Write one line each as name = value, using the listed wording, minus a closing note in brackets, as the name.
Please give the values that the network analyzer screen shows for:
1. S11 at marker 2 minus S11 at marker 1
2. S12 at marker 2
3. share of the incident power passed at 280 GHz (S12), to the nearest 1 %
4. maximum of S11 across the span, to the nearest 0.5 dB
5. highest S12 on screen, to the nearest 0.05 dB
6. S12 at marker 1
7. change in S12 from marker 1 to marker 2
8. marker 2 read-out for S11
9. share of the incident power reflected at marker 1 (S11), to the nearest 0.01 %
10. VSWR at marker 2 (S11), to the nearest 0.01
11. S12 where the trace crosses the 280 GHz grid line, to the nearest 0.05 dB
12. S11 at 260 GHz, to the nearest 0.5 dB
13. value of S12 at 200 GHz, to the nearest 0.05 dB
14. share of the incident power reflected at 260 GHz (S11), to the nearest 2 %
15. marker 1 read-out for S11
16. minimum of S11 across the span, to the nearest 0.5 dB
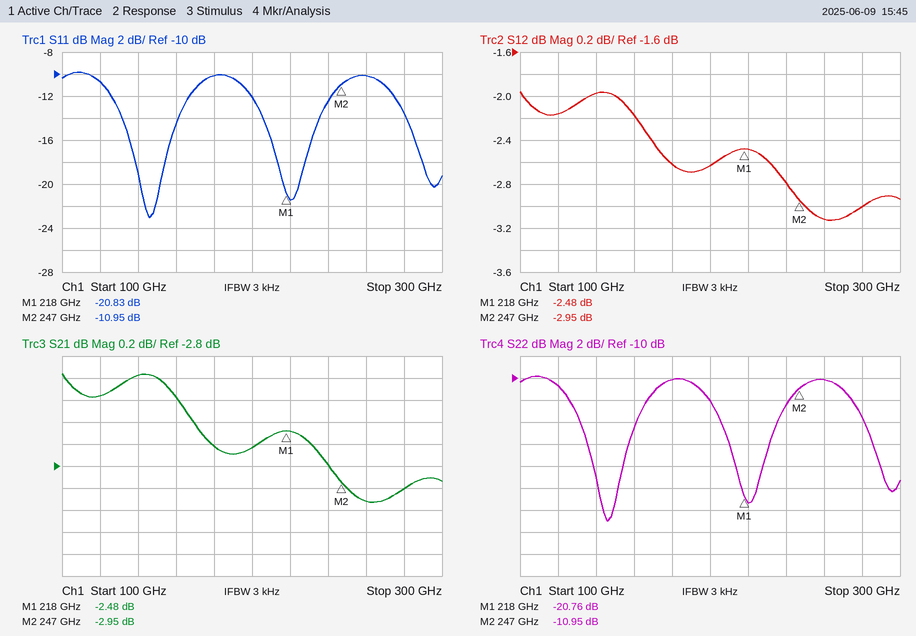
S11 at marker 2 minus S11 at marker 1 = 9.88 dB
S12 at marker 2 = -2.95 dB
share of the incident power passed at 280 GHz (S12), to the nearest 1 % = 50 %
maximum of S11 across the span, to the nearest 0.5 dB = -10.0 dB
highest S12 on screen, to the nearest 0.05 dB = -1.95 dB
S12 at marker 1 = -2.48 dB
change in S12 from marker 1 to marker 2 = -0.47 dB
marker 2 read-out for S11 = -10.95 dB
share of the incident power reflected at marker 1 (S11), to the nearest 0.01 % = 0.83 %
VSWR at marker 2 (S11), to the nearest 0.01 = 1.79
S12 where the trace crosses the 280 GHz grid line, to the nearest 0.05 dB = -3.00 dB
S11 at 260 GHz, to the nearest 0.5 dB = -10.0 dB
value of S12 at 200 GHz, to the nearest 0.05 dB = -2.65 dB
share of the incident power reflected at 260 GHz (S11), to the nearest 2 % = 10 %
marker 1 read-out for S11 = -20.83 dB
minimum of S11 across the span, to the nearest 0.5 dB = -23.0 dB
